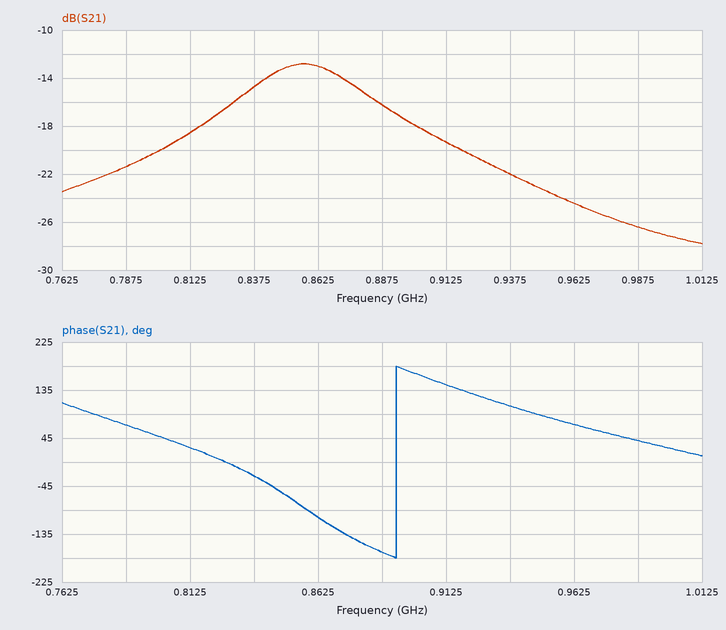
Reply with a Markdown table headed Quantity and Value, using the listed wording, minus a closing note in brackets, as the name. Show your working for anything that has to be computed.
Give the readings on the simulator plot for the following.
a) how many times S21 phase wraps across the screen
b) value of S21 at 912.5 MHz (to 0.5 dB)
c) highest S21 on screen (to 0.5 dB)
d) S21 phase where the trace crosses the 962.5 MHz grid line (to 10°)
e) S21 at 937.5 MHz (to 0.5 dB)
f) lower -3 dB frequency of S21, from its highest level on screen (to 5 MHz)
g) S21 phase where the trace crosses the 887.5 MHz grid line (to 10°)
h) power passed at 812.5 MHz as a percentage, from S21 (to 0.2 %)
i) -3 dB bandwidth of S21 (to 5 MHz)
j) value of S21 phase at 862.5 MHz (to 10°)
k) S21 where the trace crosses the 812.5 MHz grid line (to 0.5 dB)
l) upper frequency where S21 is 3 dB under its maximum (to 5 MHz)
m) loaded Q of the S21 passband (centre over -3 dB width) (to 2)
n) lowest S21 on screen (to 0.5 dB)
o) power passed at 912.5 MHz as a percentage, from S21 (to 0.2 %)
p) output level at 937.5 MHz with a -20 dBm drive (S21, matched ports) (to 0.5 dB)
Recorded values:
| Quantity | Value |
|---|---|
| how many times S21 phase wraps across the screen | 1 |
| value of S21 at 912.5 MHz | -19.5 dB |
| highest S21 on screen | -13.0 dB |
| S21 phase where the trace crosses the 962.5 MHz grid line | 70° |
| S21 at 937.5 MHz | -22.0 dB |
| lower -3 dB frequency of S21, from its highest level on screen | 830 MHz |
| S21 phase where the trace crosses the 887.5 MHz grid line | -170° |
| power passed at 812.5 MHz as a percentage, from S21 | 10^(-18.5/10) ≈ 1.4 % |
| -3 dB bandwidth of S21 | 885 MHz − 830 MHz = 55 MHz |
| value of S21 phase at 862.5 MHz | -100° |
| S21 where the trace crosses the 812.5 MHz grid line | -18.5 dB |
| upper frequency where S21 is 3 dB under its maximum | 885 MHz |
| loaded Q of the S21 passband (centre over -3 dB width) | 857.5 MHz / 55 MHz ≈ 16 |
| lowest S21 on screen | -28.0 dB |
| power passed at 912.5 MHz as a percentage, from S21 | 10^(-19.5/10) ≈ 1.12 %, so 1.2 % to the nearest 0.2 % |
| output level at 937.5 MHz with a -20 dBm drive (S21, matched ports) | -20 dBm + (-22.0 dB) = -42.0 dBm |
